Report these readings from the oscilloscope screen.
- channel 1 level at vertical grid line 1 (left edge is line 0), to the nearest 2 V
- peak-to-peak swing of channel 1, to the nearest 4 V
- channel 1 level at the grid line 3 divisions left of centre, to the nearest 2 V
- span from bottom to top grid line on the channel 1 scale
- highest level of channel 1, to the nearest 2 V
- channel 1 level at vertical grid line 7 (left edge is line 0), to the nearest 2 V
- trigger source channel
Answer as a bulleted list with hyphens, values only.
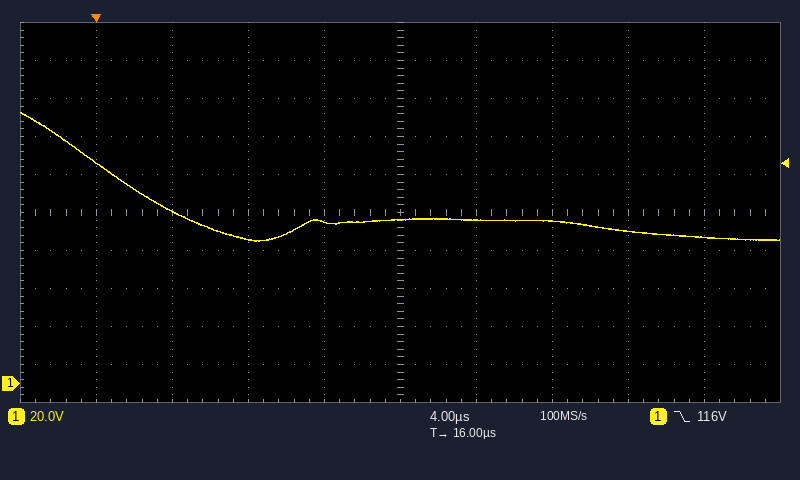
- 116 V
- 68 V
- 90 V
- 200 V
- 142 V
- 86 V
- channel 1
